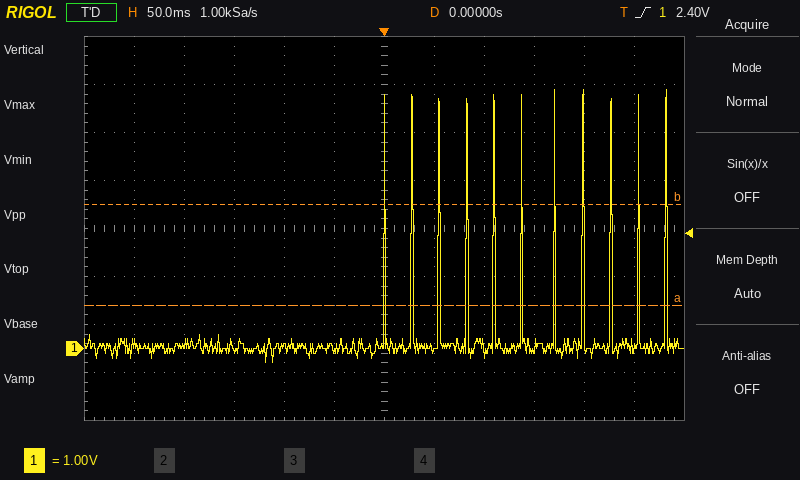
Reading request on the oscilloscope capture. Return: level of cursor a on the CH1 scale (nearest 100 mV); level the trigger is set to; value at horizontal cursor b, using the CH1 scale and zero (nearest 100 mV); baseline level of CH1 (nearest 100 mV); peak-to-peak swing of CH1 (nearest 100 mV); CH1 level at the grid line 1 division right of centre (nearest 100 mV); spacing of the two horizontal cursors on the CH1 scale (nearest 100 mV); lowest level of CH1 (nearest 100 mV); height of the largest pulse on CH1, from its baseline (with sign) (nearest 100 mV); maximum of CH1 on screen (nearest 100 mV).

900 mV
2.40 V
3.0 V
0.0 V
5.7 V
0.0 V
2.1 V
-300 mV
+5.4 V
5.4 V
